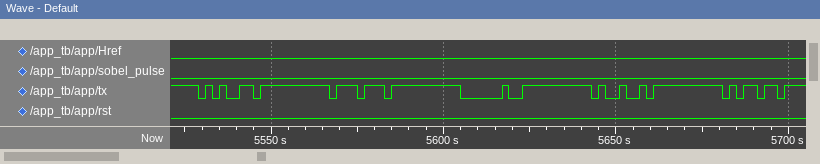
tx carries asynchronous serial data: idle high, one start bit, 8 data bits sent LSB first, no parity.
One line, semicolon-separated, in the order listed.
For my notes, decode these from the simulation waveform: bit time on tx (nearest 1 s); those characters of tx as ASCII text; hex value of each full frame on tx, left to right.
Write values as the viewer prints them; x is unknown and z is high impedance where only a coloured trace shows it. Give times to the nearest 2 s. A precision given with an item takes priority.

2 s; "ew Im"; 65, 77, 20, 49, 6D
